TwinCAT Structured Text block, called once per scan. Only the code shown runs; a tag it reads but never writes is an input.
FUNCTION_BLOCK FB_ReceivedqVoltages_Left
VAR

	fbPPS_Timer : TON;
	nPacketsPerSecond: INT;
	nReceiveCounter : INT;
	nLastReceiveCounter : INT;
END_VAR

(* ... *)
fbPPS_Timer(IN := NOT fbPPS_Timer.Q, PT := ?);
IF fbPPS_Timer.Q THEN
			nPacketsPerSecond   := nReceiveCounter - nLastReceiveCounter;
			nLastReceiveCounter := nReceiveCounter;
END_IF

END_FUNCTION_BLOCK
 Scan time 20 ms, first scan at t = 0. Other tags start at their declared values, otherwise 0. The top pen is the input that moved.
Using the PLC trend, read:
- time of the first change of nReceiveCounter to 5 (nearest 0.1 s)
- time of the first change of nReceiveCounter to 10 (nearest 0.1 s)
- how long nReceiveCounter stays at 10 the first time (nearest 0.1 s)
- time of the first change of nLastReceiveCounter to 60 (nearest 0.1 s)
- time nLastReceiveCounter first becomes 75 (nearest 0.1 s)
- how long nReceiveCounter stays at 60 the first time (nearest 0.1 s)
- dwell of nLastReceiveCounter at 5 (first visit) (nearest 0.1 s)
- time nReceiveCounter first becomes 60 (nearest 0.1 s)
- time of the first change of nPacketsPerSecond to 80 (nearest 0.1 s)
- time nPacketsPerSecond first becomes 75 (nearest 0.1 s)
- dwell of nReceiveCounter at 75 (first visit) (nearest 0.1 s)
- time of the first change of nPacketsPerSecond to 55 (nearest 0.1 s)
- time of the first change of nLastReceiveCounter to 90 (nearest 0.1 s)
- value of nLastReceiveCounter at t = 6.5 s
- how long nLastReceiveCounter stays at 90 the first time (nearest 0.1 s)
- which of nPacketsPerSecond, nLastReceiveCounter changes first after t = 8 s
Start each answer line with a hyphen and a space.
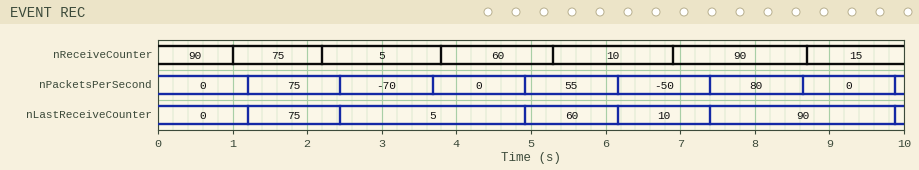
- 2.2 s
- 5.3 s
- 1.6 s
- 4.9 s
- 1.2 s
- 1.5 s
- 2.5 s
- 3.8 s
- 7.4 s
- 1.2 s
- 1.2 s
- 4.9 s
- 7.4 s
- 10
- 2.5 s
- nPacketsPerSecond
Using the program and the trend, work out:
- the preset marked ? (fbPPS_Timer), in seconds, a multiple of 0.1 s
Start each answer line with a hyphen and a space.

- 1.2 s
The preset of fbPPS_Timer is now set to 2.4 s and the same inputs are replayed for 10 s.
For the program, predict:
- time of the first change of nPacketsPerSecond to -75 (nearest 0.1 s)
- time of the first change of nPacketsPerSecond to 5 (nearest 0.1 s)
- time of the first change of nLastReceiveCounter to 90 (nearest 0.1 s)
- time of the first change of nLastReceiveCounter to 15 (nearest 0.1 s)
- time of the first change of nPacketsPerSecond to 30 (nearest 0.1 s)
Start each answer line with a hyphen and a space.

- 9.7 s
- 2.4 s
- 7.3 s
- 9.7 s
- 7.3 s
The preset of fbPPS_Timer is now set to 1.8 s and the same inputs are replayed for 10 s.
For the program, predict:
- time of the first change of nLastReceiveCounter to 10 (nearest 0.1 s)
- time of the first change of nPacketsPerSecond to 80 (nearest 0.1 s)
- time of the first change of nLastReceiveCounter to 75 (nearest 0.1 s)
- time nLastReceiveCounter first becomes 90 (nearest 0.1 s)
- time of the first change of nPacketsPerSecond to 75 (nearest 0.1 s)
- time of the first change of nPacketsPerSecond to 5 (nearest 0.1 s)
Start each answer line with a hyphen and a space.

- 5.5 s
- 7.3 s
- 1.8 s
- 7.3 s
- 1.8 s
- 5.5 s
